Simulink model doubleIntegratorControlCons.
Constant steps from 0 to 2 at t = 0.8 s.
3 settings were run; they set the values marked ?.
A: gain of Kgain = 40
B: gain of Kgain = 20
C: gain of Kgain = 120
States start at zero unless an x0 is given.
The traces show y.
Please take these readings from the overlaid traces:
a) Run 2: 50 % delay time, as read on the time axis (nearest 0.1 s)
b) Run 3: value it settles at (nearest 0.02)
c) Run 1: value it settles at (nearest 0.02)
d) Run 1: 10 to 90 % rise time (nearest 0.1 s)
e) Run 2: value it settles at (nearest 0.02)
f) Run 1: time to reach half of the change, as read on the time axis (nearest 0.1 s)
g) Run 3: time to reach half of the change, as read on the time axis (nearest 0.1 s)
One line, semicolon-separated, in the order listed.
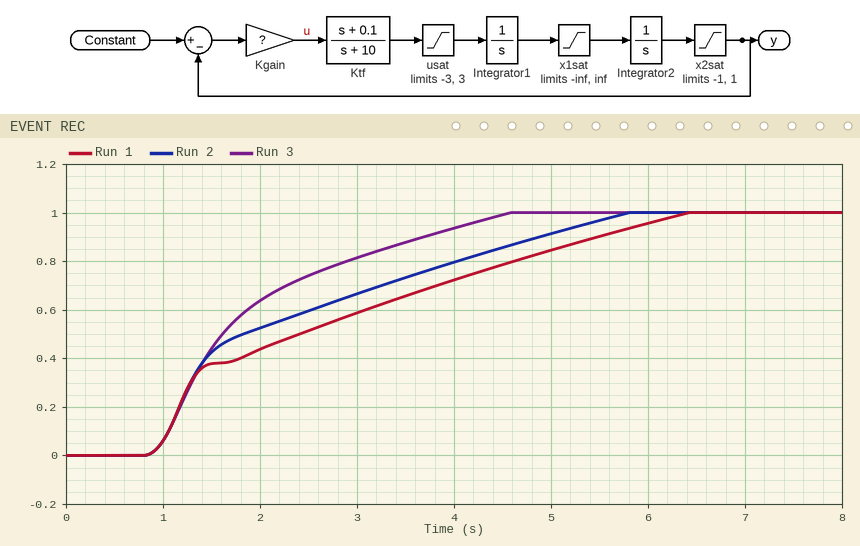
1.8 s; 1.00; 1.00; 4.4 s; 1.00; 2.4 s; 1.6 s
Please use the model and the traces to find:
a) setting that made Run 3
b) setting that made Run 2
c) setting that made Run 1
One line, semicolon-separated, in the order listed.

B; A; C
